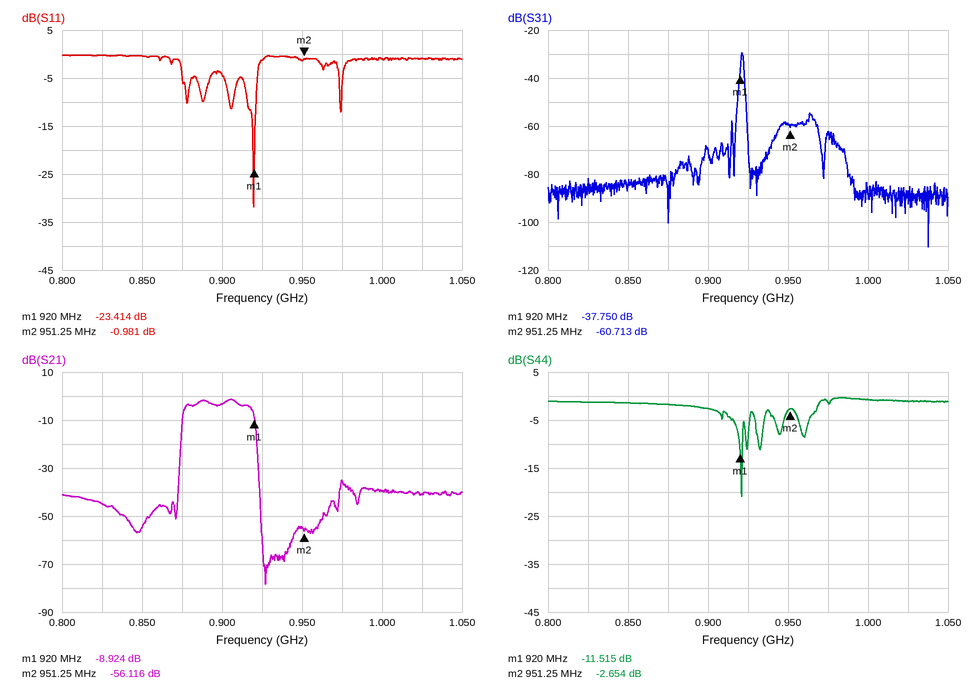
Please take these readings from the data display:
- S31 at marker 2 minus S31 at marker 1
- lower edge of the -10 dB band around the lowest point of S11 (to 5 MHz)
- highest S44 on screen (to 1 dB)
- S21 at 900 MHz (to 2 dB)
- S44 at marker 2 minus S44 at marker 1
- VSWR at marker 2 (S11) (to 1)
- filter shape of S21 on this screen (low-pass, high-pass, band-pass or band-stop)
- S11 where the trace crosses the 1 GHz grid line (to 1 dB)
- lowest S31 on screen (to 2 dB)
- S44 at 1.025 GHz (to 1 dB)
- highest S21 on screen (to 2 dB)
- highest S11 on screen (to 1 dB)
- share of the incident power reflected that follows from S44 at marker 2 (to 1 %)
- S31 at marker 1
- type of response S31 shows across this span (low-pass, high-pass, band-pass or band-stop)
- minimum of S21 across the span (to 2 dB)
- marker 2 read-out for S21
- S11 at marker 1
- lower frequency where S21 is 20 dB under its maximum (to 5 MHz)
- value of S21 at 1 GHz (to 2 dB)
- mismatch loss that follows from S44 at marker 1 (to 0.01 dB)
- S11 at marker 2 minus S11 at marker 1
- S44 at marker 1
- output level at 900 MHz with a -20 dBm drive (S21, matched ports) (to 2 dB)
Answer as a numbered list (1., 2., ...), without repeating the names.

1. -22.963 dB
2. 915 MHz
3. 0 dB
4. -4 dB
5. 8.861 dB
6. 18
7. band-pass
8. -1 dB
9. -110 dB
10. -1 dB
11. -2 dB
12. 0 dB
13. 54 %
14. -37.750 dB
15. band-pass
16. -78 dB
17. -56.116 dB
18. -23.414 dB
19. 875 MHz
20. -40 dB
21. 0.32 dB
22. 22.433 dB
23. -11.515 dB
24. -24 dBm
